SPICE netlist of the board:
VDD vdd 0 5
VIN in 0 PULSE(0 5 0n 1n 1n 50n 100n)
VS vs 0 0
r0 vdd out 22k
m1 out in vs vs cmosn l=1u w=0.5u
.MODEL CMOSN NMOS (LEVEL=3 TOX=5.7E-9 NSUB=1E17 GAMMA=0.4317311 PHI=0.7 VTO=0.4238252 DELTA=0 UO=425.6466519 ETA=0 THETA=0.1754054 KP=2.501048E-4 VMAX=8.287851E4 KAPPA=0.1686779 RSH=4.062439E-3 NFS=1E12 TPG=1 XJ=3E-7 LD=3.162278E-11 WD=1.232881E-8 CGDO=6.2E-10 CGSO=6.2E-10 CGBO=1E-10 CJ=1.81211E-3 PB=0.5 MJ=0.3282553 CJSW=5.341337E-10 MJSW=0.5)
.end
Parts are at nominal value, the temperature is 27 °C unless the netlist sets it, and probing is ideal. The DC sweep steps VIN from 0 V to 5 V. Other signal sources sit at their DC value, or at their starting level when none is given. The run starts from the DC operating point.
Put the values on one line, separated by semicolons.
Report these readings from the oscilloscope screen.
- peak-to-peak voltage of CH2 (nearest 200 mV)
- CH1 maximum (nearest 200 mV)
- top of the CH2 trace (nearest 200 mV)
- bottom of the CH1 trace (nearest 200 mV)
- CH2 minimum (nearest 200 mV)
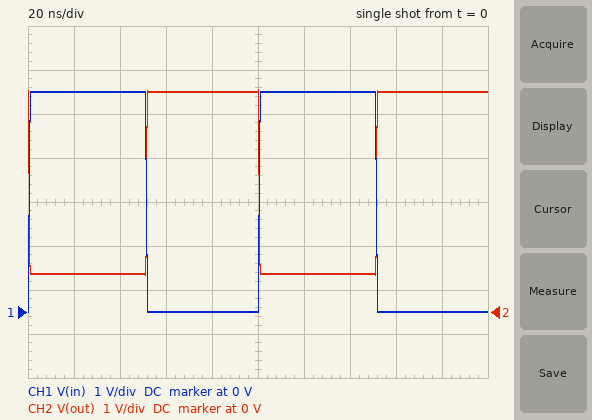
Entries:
4.2 V; 5.0 V; 5.0 V; 0 V; 800 mV
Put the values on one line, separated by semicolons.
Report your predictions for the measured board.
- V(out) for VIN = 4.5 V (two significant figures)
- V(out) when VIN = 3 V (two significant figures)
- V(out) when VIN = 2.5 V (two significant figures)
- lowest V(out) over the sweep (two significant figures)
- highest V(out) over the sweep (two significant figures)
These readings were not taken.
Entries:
960 mV; 1.8 V; 2.6 V; 860 mV; 5.0 V
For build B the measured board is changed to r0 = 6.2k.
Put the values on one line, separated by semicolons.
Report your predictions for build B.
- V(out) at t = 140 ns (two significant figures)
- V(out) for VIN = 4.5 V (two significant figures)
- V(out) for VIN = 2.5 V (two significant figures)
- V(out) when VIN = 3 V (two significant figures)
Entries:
3.1 V; 3.3 V; 4.3 V; 4.1 V
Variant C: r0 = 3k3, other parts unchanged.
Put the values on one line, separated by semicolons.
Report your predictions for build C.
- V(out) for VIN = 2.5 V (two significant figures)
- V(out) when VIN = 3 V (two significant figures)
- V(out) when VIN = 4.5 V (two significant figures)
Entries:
4.6 V; 4.5 V; 4.1 V
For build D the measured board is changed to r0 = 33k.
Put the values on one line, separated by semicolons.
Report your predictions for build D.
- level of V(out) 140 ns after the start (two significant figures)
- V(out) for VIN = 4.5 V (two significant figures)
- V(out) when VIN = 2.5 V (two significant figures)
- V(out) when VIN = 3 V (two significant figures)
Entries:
550 mV; 600 mV; 1.5 V; 970 mV
